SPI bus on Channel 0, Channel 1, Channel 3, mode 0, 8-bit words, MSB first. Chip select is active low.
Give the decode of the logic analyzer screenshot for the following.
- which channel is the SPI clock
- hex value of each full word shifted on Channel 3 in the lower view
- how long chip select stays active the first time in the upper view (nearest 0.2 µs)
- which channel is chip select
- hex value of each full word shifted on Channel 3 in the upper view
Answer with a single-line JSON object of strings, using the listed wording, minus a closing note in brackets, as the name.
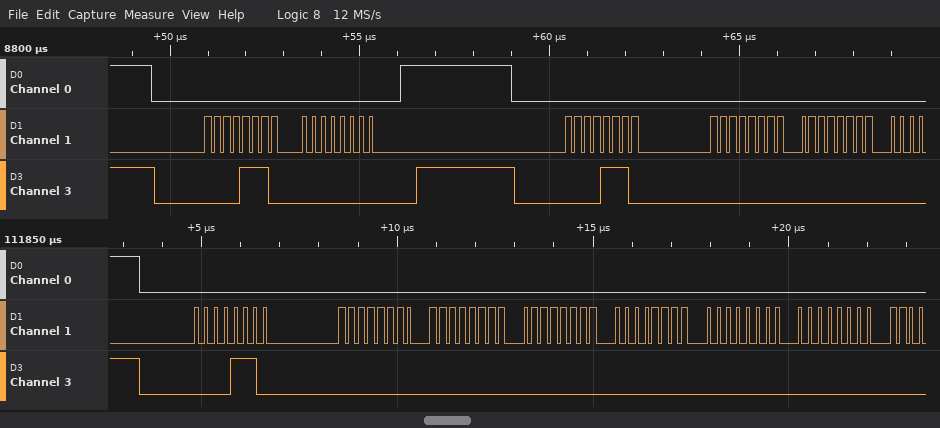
{"which channel is the SPI clock": "Channel 1", "hex value of each full word shifted on Channel 3 in the lower view": "0E, 00, 00, 00, 00, 00, 00", "how long chip select stays active the first time in the upper view": "6.6 µs", "which channel is chip select": "Channel 0", "hex value of each full word shifted on Channel 3 in the upper view": "0E, 00, 0E, 00, 00"}
